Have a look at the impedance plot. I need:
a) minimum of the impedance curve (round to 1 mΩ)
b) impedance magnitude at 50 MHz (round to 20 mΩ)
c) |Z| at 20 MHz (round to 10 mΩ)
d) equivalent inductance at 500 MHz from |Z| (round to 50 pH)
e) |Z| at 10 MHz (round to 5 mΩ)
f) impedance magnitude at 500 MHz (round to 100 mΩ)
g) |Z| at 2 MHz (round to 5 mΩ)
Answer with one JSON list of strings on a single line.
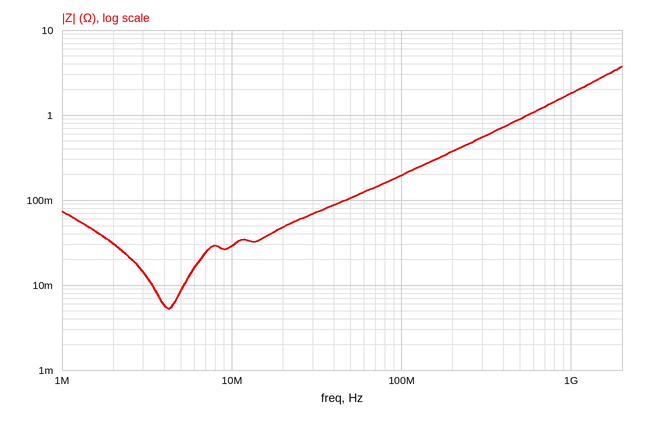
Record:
["5 mΩ", "100 mΩ", "50 mΩ", "300 pH", "30 mΩ", "900 mΩ", "30 mΩ"]
